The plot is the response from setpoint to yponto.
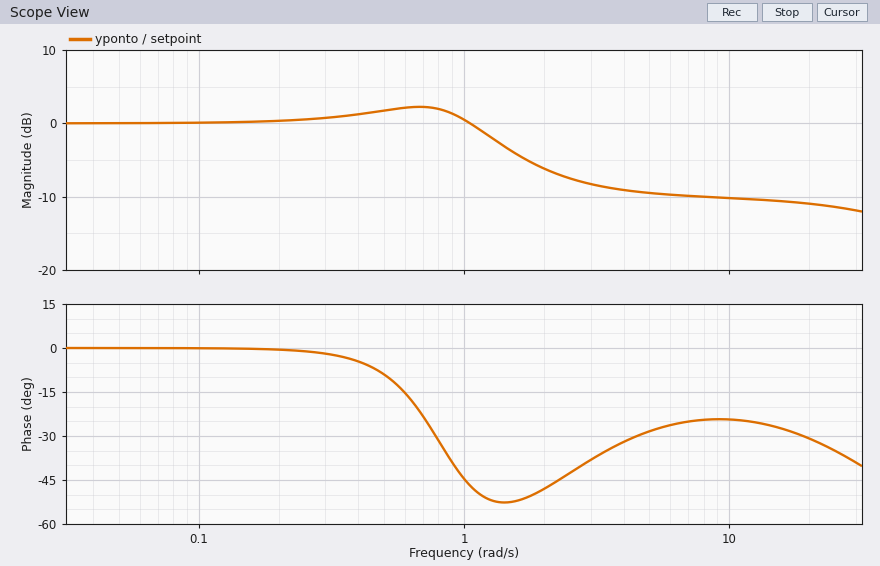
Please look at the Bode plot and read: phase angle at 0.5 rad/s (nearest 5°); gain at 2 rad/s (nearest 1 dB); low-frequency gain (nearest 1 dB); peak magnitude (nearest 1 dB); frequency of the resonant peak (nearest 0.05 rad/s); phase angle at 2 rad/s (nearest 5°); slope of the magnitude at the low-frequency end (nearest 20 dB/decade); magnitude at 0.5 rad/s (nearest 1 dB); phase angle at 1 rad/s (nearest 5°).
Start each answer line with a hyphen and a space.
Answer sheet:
- -10°
- -6 dB
- 0 dB
- 2 dB
- 0.65 rad/s
- -50°
- 0 dB/decade
- 2 dB
- -45°
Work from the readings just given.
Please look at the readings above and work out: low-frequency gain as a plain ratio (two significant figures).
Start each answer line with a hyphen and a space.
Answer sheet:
- 1.0
